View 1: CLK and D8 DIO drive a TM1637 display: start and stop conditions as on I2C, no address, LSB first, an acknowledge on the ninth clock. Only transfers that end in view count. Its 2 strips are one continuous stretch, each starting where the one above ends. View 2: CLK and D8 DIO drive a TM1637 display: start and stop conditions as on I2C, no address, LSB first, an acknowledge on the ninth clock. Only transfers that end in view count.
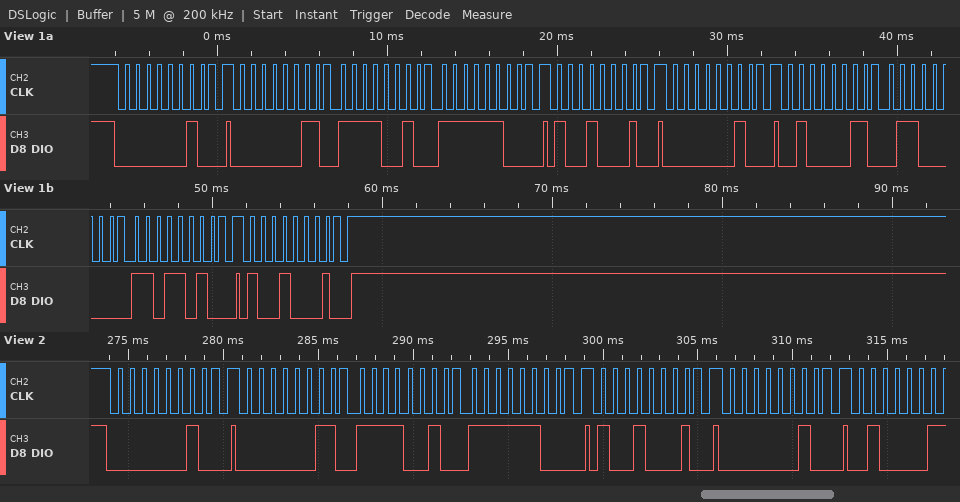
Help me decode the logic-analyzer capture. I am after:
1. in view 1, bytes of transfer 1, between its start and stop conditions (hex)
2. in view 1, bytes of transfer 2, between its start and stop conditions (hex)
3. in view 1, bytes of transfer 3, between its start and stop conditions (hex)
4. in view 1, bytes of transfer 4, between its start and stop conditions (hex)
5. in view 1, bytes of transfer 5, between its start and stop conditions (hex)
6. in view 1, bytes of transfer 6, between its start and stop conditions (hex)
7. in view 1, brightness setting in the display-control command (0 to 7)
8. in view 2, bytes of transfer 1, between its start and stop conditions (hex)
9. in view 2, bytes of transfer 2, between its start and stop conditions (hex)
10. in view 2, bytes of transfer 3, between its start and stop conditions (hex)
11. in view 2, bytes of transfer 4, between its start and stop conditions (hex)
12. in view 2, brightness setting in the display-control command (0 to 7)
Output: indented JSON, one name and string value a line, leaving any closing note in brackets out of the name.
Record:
{
  "in view 1, bytes of transfer 1, between its start and stop conditions": "40",
  "in view 1, bytes of transfer 2, between its start and stop conditions": "C0 4F 3F",
  "in view 1, bytes of transfer 3, between its start and stop conditions": "89",
  "in view 1, bytes of transfer 4, between its start and stop conditions": "40",
  "in view 1, bytes of transfer 5, between its start and stop conditions": "C2 06 5B",
  "in view 1, bytes of transfer 6, between its start and stop conditions": "89",
  "in view 1, brightness setting in the display-control command": "1",
  "in view 2, bytes of transfer 1, between its start and stop conditions": "40",
  "in view 2, bytes of transfer 2, between its start and stop conditions": "C0 4F 3F",
  "in view 2, bytes of transfer 3, between its start and stop conditions": "89",
  "in view 2, bytes of transfer 4, between its start and stop conditions": "40",
  "in view 2, brightness setting in the display-control command": "1"
}
